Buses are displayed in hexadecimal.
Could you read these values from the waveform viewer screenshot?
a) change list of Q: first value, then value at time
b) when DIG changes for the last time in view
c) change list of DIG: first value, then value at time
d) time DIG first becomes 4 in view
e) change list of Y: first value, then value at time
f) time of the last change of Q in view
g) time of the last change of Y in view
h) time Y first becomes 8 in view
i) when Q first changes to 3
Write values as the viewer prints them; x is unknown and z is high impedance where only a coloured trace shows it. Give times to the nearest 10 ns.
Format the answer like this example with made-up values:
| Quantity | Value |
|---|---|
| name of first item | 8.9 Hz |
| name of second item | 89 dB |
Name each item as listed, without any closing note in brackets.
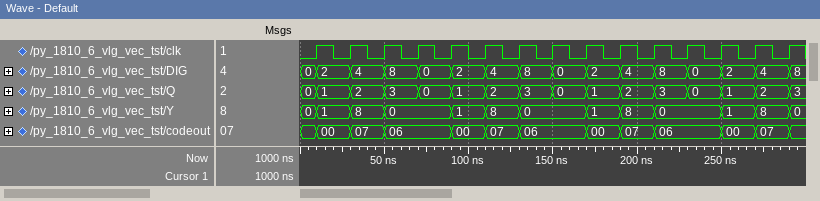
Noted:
| Quantity | Value |
|---|---|
| change list of Q: first value, then value at time | 0, 1 at 10 ns, 2 at 30 ns, 3 at 50 ns, 0 at 70 ns, 1 at 90 ns, 2 at 110 ns, 3 at 130 ns, 0 at 150 ns, 1 at 170 ns, 2 at 190 ns, 3 at 210 ns, 0 at 230 ns, 1 at 250 ns, 2 at 270 ns, 3 at 290 ns |
| when DIG changes for the last time in view | 290 ns |
| change list of DIG: first value, then value at time | 0, 2 at 10 ns, 4 at 30 ns, 8 at 50 ns, 0 at 70 ns, 2 at 90 ns, 4 at 110 ns, 8 at 130 ns, 0 at 150 ns, 2 at 170 ns, 4 at 190 ns, 8 at 210 ns, 0 at 230 ns, 2 at 250 ns, 4 at 270 ns, 8 at 290 ns |
| time DIG first becomes 4 in view | 30 ns |
| change list of Y: first value, then value at time | 0, 1 at 10 ns, 8 at 30 ns, 0 at 50 ns, 1 at 90 ns, 8 at 110 ns, 0 at 130 ns, 1 at 170 ns, 8 at 190 ns, 0 at 210 ns, 1 at 250 ns, 8 at 270 ns, 0 at 290 ns |
| time of the last change of Q in view | 290 ns |
| time of the last change of Y in view | 290 ns |
| time Y first becomes 8 in view | 30 ns |
| when Q first changes to 3 | 50 ns |
